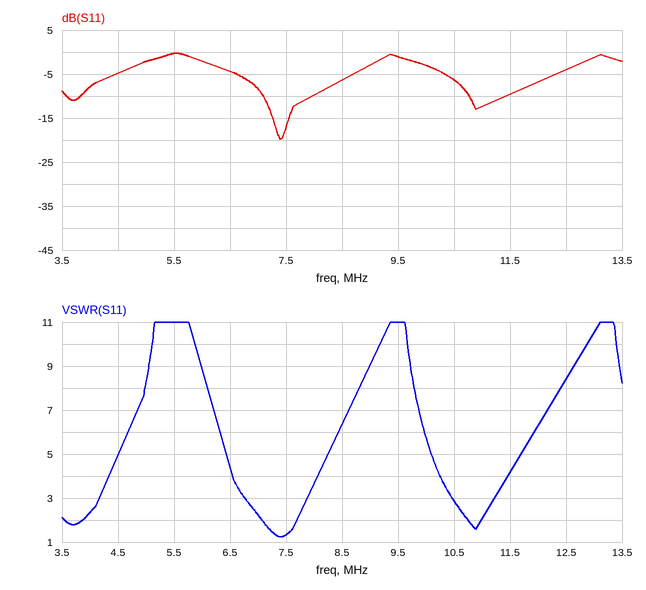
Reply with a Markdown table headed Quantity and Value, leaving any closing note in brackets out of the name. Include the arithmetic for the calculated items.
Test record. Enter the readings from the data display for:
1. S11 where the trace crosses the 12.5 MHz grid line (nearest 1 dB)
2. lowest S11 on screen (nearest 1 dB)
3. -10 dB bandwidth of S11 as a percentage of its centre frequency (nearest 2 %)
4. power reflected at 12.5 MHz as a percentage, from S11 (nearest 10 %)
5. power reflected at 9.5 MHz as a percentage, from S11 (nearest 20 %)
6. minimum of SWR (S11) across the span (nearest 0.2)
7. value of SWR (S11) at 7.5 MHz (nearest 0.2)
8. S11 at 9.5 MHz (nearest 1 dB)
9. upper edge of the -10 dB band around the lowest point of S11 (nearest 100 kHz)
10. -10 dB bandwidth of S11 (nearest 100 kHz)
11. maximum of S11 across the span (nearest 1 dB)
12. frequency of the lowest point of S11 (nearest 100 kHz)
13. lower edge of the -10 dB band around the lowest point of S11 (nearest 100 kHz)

| Quantity | Value |
|---|---|
| S11 where the trace crosses the 12.5 MHz grid line | -4 dB |
| lowest S11 on screen | -20 dB |
| -10 dB bandwidth of S11 as a percentage of its centre frequency | 900 kHz / 7.55 MHz ≈ 12 % |
| power reflected at 12.5 MHz as a percentage, from S11 | 10^(-4/10) ≈ 40 % |
| power reflected at 9.5 MHz as a percentage, from S11 | 10^(-1/10) ≈ 79.4 %, so 80 % to the nearest 20 % |
| minimum of SWR (S11) across the span | 1.2 |
| value of SWR (S11) at 7.5 MHz | 1.4 |
| S11 at 9.5 MHz | -1 dB |
| upper edge of the -10 dB band around the lowest point of S11 | 8.0 MHz |
| -10 dB bandwidth of S11 | 8.0 MHz − 7.1 MHz = 900 kHz |
| maximum of S11 across the span | 0 dB |
| frequency of the lowest point of S11 | 7.4 MHz |
| lower edge of the -10 dB band around the lowest point of S11 | 7.1 MHz |
